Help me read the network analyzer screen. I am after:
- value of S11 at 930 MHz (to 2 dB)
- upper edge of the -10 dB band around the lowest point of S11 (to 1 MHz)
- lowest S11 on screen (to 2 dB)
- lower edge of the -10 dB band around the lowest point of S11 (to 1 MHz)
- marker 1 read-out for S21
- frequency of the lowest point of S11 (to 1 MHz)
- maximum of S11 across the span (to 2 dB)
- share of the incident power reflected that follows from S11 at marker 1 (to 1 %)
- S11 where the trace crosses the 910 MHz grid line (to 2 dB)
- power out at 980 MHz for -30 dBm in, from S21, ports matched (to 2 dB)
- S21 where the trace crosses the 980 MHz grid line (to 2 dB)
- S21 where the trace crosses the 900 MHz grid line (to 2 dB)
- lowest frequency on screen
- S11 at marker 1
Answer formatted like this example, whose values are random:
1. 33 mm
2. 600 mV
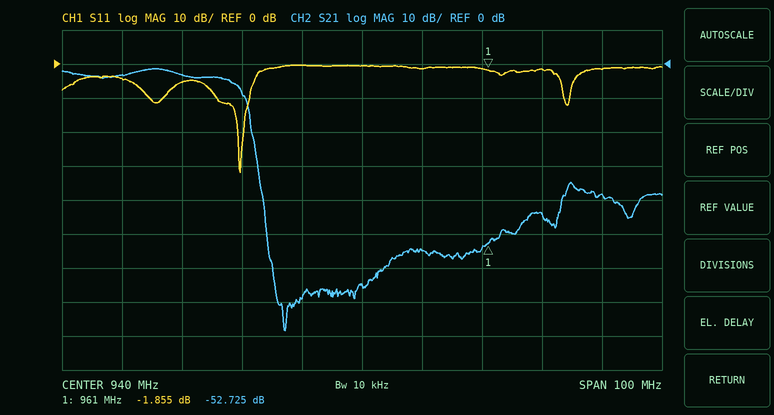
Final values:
1. 0 dB
2. 921 MHz
3. -32 dB
4. 916 MHz
5. -52.725 dB
6. 920 MHz
7. 0 dB
8. 65 %
9. -6 dB
10. -68 dBm
11. -38 dB
12. -4 dB
13. 890 MHz
14. -1.855 dB
